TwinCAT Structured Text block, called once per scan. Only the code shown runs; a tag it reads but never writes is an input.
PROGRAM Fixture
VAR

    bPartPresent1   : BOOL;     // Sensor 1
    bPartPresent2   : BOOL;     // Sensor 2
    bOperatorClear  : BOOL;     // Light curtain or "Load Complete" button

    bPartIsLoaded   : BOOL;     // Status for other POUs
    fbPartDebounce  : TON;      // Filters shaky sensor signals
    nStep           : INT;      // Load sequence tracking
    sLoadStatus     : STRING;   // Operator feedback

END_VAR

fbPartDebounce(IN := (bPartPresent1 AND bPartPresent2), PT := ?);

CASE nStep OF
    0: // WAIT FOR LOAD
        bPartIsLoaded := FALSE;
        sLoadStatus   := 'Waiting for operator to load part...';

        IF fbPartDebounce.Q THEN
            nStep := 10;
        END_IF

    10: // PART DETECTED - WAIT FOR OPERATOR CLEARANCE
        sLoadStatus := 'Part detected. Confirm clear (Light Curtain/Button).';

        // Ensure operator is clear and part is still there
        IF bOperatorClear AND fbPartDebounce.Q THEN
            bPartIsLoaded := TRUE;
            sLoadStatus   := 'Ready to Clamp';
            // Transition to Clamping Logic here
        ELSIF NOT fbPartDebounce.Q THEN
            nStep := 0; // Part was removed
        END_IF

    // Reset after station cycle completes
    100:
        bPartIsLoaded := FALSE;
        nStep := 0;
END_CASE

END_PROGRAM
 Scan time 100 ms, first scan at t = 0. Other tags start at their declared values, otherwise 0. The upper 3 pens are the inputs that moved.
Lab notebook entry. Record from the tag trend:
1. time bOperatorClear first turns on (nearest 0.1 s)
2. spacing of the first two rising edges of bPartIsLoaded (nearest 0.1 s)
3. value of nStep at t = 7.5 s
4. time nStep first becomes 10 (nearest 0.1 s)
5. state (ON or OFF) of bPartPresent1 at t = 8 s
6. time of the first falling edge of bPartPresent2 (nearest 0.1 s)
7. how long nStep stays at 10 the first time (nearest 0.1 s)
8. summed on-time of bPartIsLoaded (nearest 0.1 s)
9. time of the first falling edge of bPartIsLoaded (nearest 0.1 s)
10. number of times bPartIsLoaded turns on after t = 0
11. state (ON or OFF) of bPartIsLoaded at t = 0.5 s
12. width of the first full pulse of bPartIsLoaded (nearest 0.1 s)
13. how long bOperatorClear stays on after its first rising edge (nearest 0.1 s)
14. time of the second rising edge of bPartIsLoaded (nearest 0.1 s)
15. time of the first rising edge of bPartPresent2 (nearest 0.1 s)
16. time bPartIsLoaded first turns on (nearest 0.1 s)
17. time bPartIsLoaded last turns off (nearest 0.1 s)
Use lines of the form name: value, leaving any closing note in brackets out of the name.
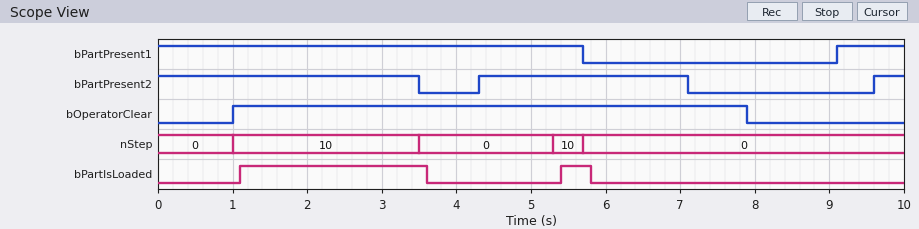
time bOperatorClear first turns on: 1.0 s
spacing of the first two rising edges of bPartIsLoaded: 4.3 s
value of nStep at t = 7.5 s: 0
time nStep first becomes 10: 1.0 s
state (ON or OFF) of bPartPresent1 at t = 8 s: OFF
time of the first falling edge of bPartPresent2: 3.5 s
how long nStep stays at 10 the first time: 2.5 s
summed on-time of bPartIsLoaded: 2.9 s
time of the first falling edge of bPartIsLoaded: 3.6 s
number of times bPartIsLoaded turns on after t = 0: 2
state (ON or OFF) of bPartIsLoaded at t = 0.5 s: OFF
width of the first full pulse of bPartIsLoaded: 2.5 s
how long bOperatorClear stays on after its first rising edge: 6.9 s
time of the second rising edge of bPartIsLoaded: 5.4 s
time of the first rising edge of bPartPresent2: 4.3 s
time bPartIsLoaded first turns on: 1.1 s
time bPartIsLoaded last turns off: 5.8 s
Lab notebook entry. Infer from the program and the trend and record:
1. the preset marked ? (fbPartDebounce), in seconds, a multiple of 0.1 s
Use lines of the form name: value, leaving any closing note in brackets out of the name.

the preset marked ? (fbPartDebounce), in seconds, a multiple of 0.1 s: 1.0 s
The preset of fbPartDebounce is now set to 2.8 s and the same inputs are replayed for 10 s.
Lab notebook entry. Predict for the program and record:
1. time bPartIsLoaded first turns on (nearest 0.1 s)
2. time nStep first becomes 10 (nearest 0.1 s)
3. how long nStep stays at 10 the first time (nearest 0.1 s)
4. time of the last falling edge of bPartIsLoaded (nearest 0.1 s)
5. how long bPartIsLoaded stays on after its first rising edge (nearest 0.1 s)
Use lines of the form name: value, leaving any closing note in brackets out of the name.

time bPartIsLoaded first turns on: 2.9 s
time nStep first becomes 10: 2.8 s
how long nStep stays at 10 the first time: 0.7 s
time of the last falling edge of bPartIsLoaded: 3.6 s
how long bPartIsLoaded stays on after its first rising edge: 0.7 s
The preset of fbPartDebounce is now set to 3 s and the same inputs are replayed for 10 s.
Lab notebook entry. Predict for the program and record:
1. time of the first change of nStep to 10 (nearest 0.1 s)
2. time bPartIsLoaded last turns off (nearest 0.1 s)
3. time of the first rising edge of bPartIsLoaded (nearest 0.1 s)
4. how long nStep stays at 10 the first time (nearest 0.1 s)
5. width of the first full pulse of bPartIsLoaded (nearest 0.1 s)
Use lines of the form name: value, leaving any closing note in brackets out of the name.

time of the first change of nStep to 10: 3.0 s
time bPartIsLoaded last turns off: 3.6 s
time of the first rising edge of bPartIsLoaded: 3.1 s
how long nStep stays at 10 the first time: 0.5 s
width of the first full pulse of bPartIsLoaded: 0.5 s
